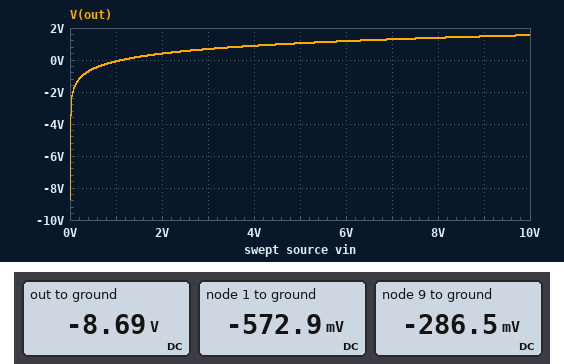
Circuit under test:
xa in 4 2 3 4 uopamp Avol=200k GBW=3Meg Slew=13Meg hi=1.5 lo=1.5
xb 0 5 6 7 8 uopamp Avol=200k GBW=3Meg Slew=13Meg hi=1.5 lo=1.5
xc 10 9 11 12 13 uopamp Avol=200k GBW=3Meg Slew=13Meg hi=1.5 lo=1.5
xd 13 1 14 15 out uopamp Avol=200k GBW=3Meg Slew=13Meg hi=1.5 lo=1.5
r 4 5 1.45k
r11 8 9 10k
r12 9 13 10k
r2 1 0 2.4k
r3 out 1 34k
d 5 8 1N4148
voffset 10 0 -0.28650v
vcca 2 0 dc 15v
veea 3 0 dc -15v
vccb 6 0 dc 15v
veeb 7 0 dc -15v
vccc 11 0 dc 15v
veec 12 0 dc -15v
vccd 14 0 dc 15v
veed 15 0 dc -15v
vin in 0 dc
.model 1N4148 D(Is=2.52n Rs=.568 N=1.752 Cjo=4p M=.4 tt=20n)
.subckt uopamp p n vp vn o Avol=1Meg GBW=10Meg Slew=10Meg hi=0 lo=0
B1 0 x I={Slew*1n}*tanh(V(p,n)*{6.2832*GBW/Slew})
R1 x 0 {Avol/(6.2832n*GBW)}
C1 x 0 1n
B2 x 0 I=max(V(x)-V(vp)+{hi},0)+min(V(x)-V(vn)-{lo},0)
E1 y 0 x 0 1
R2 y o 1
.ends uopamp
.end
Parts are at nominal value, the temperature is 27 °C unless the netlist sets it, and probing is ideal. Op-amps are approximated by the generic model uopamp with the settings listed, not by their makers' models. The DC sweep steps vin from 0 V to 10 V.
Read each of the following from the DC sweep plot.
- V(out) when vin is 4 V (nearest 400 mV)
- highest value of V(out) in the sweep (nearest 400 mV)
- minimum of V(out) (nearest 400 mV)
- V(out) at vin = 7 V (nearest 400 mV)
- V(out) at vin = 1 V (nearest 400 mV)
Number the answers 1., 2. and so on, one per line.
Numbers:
1. 800 mV
2. 1.6 V
3. -8.8 V
4. 1.2 V
5. 0 V
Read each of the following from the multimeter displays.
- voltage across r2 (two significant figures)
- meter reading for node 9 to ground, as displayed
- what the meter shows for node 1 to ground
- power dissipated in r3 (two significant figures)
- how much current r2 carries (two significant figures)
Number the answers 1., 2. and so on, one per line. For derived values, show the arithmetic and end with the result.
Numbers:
1. 0 V - (-572.9 mV) = 570 mV
2. -286.5 mV
3. -572.9 mV
4. (-572.9 mV - (-8.69 V))^2 / 34 kΩ = 1.9 mW
5. (0 V - (-572.9 mV)) / 2.4 kΩ = 240 µA
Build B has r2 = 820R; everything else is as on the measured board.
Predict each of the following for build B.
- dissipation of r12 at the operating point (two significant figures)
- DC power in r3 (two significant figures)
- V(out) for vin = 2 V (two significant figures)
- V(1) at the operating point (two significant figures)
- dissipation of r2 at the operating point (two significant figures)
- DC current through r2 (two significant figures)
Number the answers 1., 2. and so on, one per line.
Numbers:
1. 8.2 µW
2. 5.1 mW
3. 1.1 V
4. -320 mV
5. 120 µW
6. 390 µA
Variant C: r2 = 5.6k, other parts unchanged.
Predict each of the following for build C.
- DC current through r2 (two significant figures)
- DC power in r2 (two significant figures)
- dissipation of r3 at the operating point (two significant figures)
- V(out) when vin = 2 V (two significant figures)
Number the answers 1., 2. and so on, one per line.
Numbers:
1. 100 µA
2. 59 µW
3. 360 µW
4. 190 mV
